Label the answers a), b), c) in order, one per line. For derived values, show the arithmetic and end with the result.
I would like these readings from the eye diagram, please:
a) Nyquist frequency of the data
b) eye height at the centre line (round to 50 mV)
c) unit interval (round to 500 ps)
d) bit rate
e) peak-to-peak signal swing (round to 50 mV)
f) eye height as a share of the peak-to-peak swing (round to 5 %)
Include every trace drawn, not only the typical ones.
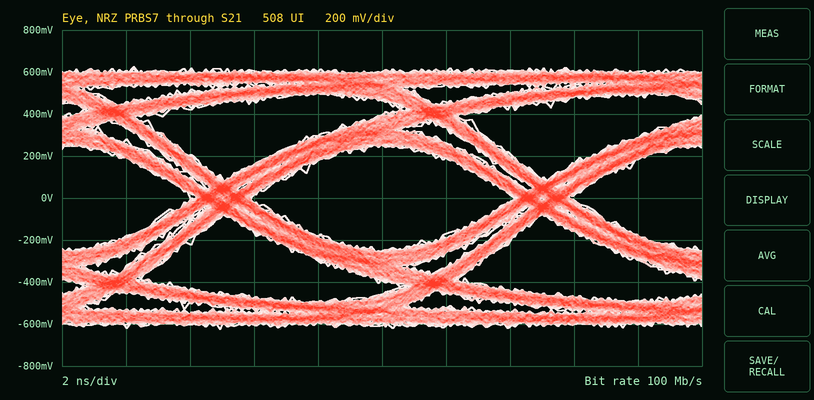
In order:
a) 50 MHz
b) 500 mV
c) 10.0 ns
d) 100 Mb/s
e) 1.25 V
f) 500 mV / 1.25 V ≈ 40 %
